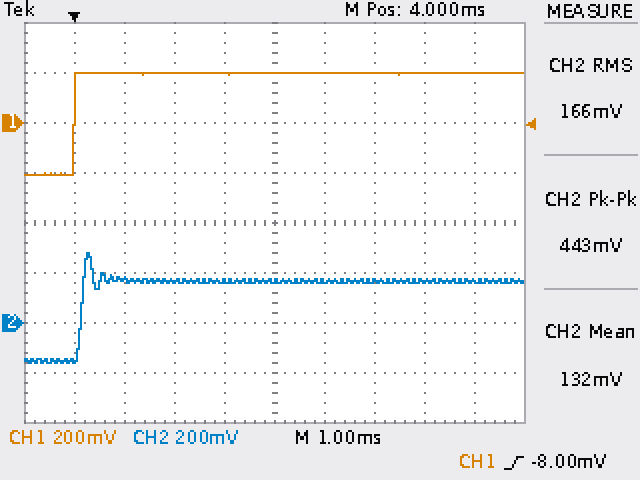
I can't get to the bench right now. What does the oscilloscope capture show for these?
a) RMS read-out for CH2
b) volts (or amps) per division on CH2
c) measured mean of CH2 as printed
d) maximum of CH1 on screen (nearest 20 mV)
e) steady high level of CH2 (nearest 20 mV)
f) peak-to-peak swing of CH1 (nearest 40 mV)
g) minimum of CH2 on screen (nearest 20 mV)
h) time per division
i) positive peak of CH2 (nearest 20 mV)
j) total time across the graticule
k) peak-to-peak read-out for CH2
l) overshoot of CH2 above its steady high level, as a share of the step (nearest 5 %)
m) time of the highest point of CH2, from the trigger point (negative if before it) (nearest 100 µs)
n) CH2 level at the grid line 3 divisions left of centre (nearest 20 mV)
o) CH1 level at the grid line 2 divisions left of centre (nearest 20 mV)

166 mV
200 mV
132 mV
200 mV
160 mV
400 mV
-160 mV
1 ms
280 mV
10 ms
443 mV
35 %
+300 µs
180 mV
200 mV
